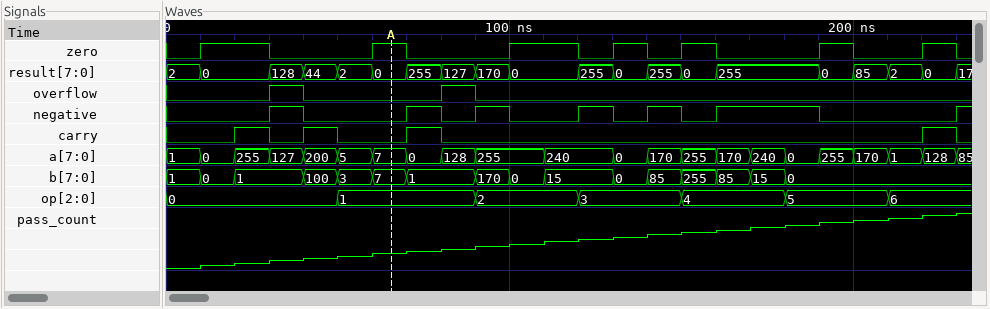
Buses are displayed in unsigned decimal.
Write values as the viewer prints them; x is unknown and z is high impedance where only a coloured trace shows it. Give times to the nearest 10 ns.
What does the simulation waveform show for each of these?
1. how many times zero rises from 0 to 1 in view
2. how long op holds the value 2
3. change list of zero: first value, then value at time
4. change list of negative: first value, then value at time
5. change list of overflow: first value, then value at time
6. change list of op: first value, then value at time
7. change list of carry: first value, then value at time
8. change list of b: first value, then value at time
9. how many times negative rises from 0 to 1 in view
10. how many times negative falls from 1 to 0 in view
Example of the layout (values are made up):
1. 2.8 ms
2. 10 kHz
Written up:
1. 7
2. 30 ns
3. 0, 1 at 10 ns, 0 at 30 ns, 1 at 60 ns, 0 at 70 ns, 1 at 100 ns, 0 at 120 ns, 1 at 130 ns, 0 at 140 ns, 1 at 150 ns, 0 at 160 ns, 1 at 190 ns, 0 at 200 ns, 1 at 220 ns, 0 at 230 ns
4. 0, 1 at 30 ns, 0 at 40 ns, 1 at 70 ns, 0 at 80 ns, 1 at 90 ns, 0 at 100 ns, 1 at 120 ns, 0 at 130 ns, 1 at 140 ns, 0 at 150 ns, 1 at 160 ns, 0 at 190 ns, 1 at 230 ns
5. 0, 1 at 30 ns, 0 at 40 ns, 1 at 80 ns, 0 at 90 ns
6. 0, 1 at 50 ns, 2 at 90 ns, 3 at 120 ns, 4 at 150 ns, 5 at 180 ns, 6 at 210 ns
7. 0, 1 at 20 ns, 0 at 30 ns, 1 at 40 ns, 0 at 50 ns, 1 at 70 ns, 0 at 80 ns, 1 at 220 ns, 0 at 230 ns
8. 1, 0 at 10 ns, 1 at 20 ns, 100 at 40 ns, 3 at 50 ns, 7 at 60 ns, 1 at 70 ns, 170 at 90 ns, 0 at 100 ns, 15 at 110 ns, 0 at 130 ns, 85 at 140 ns, 255 at 150 ns, 85 at 160 ns, 15 at 170 ns, 0 at 180 ns
9. 7
10. 6
